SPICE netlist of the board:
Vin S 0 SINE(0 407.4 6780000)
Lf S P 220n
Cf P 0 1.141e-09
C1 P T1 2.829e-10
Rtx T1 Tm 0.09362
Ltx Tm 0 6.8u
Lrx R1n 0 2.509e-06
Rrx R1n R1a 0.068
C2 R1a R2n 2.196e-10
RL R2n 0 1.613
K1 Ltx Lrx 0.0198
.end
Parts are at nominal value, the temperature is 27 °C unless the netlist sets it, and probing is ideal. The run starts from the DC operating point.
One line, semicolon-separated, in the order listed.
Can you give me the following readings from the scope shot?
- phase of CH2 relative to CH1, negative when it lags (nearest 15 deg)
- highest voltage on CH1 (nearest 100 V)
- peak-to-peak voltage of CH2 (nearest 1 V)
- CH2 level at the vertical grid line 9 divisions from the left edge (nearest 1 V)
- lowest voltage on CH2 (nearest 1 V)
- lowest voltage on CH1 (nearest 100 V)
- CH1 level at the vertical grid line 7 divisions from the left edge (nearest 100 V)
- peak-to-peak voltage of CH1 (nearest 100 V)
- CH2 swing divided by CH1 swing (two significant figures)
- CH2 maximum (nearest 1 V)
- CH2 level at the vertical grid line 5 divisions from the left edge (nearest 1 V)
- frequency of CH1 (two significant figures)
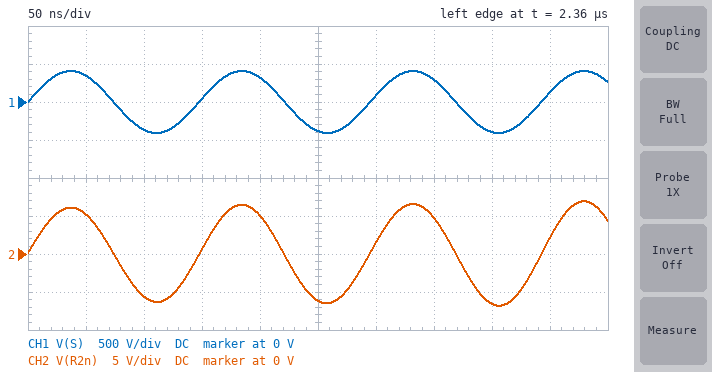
0 deg; 400 V; 14 V; 2 V; -7 V; -400 V; 300 V; 800 V; 0.017; 7 V; -6 V; 6.8 MHz
